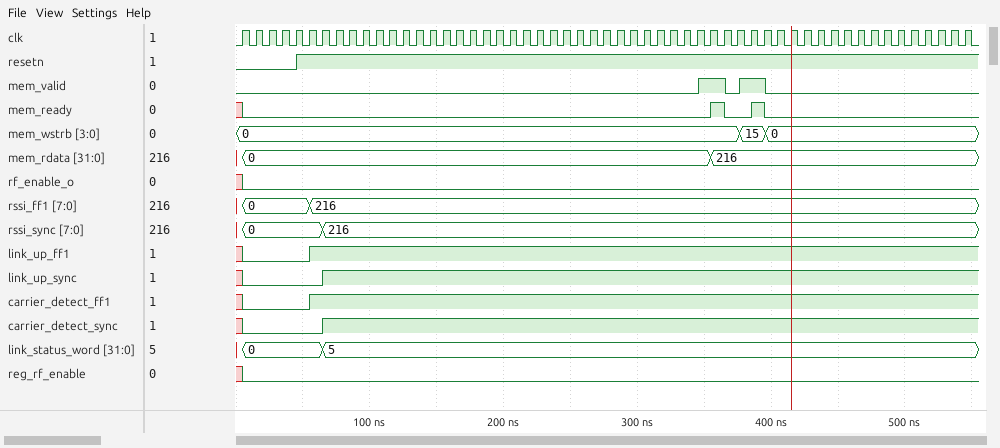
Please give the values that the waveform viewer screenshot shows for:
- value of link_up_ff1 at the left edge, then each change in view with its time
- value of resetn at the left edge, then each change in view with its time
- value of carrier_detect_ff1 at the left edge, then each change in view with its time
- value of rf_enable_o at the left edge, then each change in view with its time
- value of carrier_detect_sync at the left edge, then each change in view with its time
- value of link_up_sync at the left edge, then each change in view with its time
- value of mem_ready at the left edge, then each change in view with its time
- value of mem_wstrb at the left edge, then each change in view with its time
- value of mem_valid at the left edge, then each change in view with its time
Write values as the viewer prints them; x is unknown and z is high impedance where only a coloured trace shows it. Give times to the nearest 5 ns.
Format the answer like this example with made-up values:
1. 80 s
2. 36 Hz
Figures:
1. x, 0 at 5 ns, 1 at 55 ns
2. 0, 1 at 45 ns
3. x, 0 at 5 ns, 1 at 55 ns
4. x, 0 at 5 ns
5. x, 0 at 5 ns, 1 at 65 ns
6. x, 0 at 5 ns, 1 at 65 ns
7. x, 0 at 5 ns, 1 at 355 ns, 0 at 365 ns, 1 at 385 ns, 0 at 395 ns
8. 0, 15 at 375 ns, 0 at 395 ns
9. 0, 1 at 345 ns, 0 at 365 ns, 1 at 375 ns, 0 at 395 ns
